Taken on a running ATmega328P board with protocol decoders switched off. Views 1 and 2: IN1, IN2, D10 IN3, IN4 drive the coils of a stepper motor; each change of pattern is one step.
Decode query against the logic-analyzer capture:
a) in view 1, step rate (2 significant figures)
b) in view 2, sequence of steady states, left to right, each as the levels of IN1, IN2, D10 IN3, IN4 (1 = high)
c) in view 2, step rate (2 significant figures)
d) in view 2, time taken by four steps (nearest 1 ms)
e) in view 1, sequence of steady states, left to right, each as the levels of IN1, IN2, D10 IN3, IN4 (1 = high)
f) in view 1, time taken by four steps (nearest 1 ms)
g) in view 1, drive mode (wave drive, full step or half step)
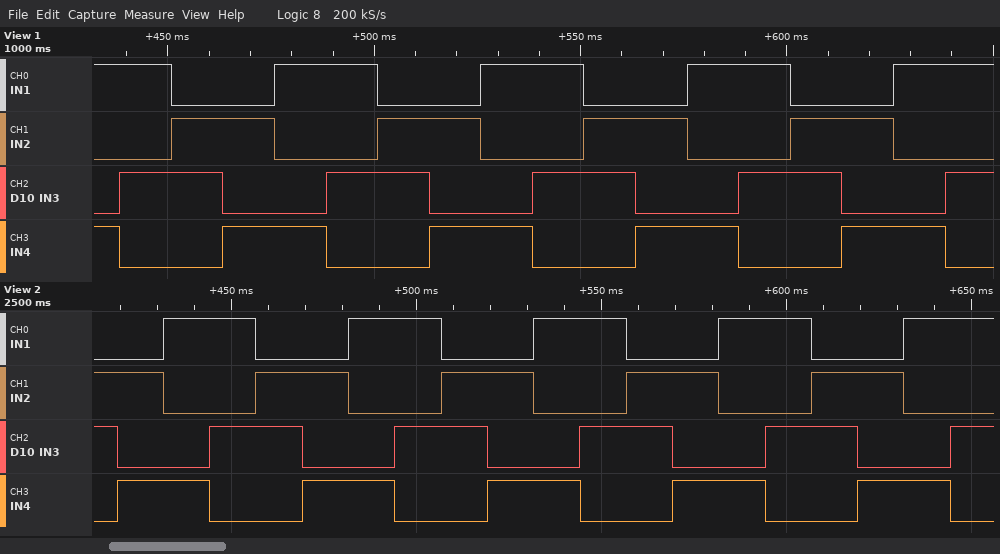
80 steps/s
0110 0101 1001 1010 0110 0101 1001 1010 0110 0101 1001 1010 0110 0101 1001 1010 0110 0101 1001 1010
80 steps/s
50 ms
1001 1010 0110 0101 1001 1010 0110 0101 1001 1010 0110 0101 1001 1010 0110 0101 1001 1010
50 ms
full step
